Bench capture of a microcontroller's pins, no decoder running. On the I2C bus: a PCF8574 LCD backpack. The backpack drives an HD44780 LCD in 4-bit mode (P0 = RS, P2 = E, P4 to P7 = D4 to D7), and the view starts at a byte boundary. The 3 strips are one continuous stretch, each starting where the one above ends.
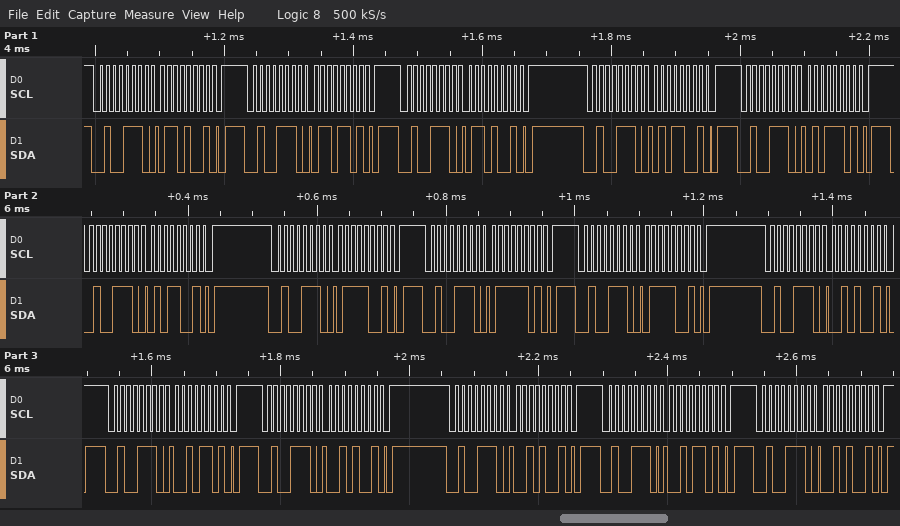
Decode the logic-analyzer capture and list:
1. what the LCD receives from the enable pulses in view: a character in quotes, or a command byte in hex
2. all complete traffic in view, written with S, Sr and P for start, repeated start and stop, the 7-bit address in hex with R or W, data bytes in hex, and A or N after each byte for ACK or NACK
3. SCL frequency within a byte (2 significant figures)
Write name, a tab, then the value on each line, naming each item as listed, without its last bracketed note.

what the LCD receives from the enable pulses in view: a character in quotes, or a command byte in hex	'e' 'r'
all complete traffic in view, written with S, Sr and P for start, repeated start and stop, the 7-bit address in hex with R or W, data bytes in hex, and A or N after each byte for ACK or NACK	S 27W A 69 A P S 27W A 6D A P S 27W A 69 A P S 27W A 59 A P S 27W A 5D A P S 27W A 59 A P S 27W A 79 A P S 27W A 7D A P S 27W A 79 A P S 27W A 29 A P S 27W A 2D A P S 27W A 29 A P S 27W A 29 A P S 27W A 2D A P S 27W A 29 A P
SCL frequency within a byte	100 kHz
